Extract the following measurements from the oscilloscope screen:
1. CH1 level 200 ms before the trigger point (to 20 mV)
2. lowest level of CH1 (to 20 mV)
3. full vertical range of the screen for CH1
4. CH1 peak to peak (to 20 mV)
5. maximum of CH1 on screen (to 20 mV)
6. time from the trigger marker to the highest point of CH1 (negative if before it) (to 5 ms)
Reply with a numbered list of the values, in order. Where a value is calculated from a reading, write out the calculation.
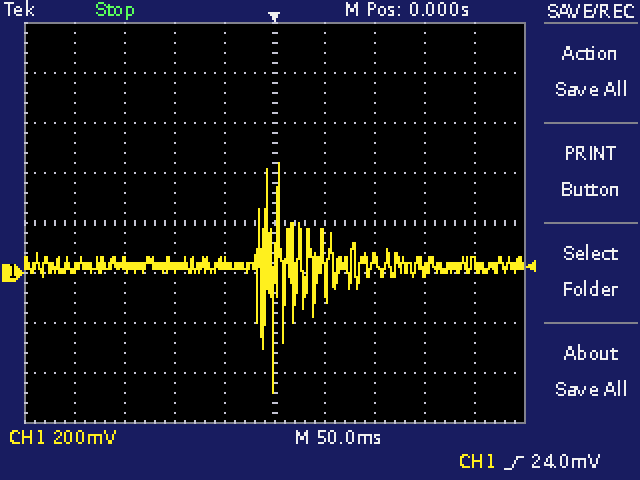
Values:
1. 20 mV
2. -480 mV
3. 1.6 V
4. 440 mV − (-480 mV) = 920 mV
5. 440 mV
6. +5 ms
